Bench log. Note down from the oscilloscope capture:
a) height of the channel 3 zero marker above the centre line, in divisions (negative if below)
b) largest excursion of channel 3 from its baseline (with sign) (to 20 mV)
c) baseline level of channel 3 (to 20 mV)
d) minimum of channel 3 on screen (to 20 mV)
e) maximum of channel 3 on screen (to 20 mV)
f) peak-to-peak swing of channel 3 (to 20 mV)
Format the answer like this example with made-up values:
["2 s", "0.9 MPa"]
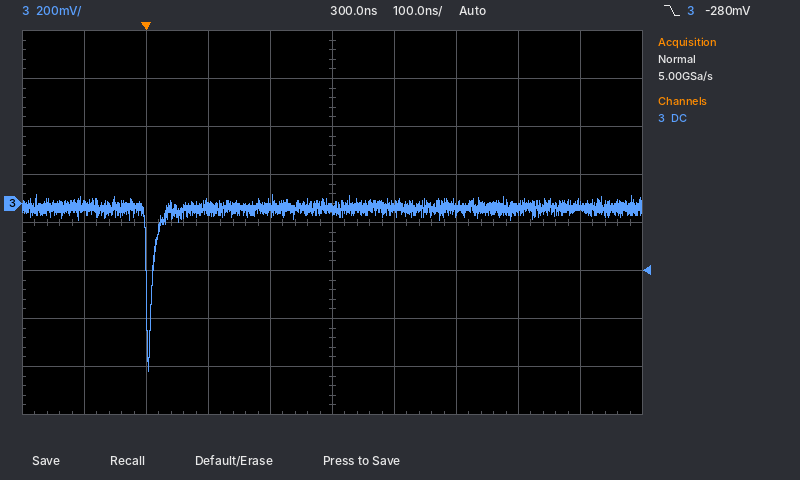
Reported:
["+0.4 div", "-680 mV", "-20 mV", "-700 mV", "40 mV", "740 mV"]
